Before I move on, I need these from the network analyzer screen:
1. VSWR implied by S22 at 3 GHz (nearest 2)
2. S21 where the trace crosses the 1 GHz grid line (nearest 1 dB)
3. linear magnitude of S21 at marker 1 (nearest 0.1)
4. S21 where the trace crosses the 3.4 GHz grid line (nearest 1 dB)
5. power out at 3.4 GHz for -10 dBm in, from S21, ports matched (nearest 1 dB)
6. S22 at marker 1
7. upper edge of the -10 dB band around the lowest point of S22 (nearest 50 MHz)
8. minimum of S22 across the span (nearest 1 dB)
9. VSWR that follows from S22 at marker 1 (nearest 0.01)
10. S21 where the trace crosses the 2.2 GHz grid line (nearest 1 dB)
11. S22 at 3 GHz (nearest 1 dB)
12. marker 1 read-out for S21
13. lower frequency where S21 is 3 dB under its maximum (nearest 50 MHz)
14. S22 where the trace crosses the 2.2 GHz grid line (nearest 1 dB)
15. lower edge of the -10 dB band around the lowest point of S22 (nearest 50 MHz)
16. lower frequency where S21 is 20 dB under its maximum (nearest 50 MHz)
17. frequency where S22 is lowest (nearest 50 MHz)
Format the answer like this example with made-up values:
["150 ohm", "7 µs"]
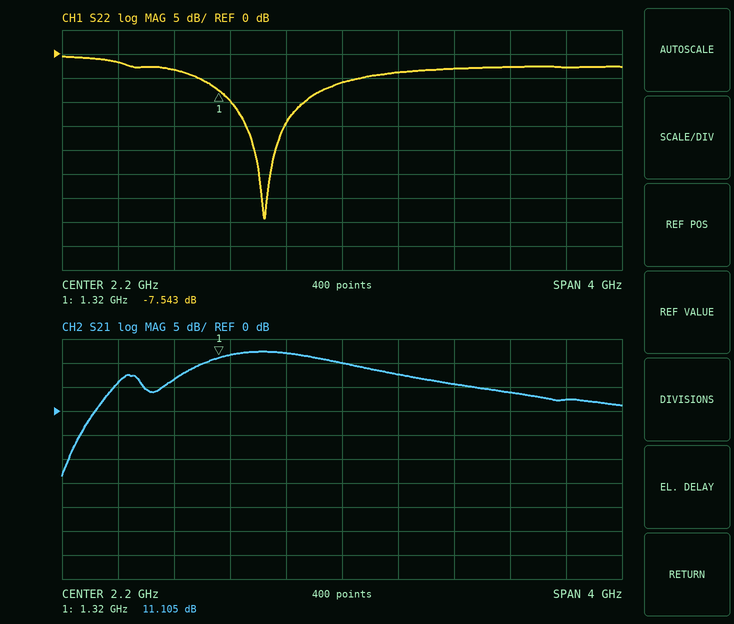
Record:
["6", "7 dB", "3.6", "4 dB", "-6 dBm", "-7.543 dB", "1.95 GHz", "-34 dB", "2.45", "10 dB", "-3 dB", "11.105 dB", "1.15 GHz", "-6 dB", "1.40 GHz", "300 MHz", "1.65 GHz"]
